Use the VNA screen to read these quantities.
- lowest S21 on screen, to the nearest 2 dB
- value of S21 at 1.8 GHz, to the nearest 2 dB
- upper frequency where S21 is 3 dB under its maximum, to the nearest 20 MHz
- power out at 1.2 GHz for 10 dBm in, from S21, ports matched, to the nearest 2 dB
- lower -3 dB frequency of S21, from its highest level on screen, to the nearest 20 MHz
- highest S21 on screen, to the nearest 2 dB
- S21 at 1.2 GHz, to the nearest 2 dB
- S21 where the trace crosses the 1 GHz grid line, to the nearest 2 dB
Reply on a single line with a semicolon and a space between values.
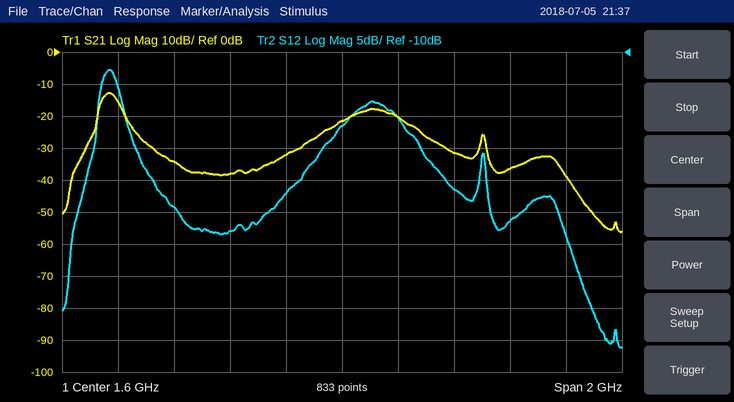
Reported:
-56 dB; -20 dB; 800 MHz; -28 dBm; 740 MHz; -12 dB; -38 dB; -34 dB
